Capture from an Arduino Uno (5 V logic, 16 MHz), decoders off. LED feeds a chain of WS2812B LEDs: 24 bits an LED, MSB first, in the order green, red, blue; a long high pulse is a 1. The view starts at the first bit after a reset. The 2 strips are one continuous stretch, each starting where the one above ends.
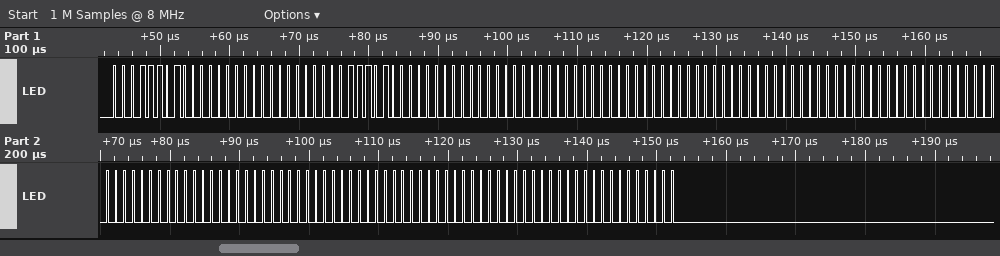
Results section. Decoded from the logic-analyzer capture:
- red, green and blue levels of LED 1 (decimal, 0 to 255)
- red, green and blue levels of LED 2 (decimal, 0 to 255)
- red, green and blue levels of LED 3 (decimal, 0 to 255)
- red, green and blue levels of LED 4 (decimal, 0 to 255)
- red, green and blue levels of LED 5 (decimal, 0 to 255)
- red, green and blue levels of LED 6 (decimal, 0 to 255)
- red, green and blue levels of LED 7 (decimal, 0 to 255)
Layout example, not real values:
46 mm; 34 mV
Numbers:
0, 29, 0; 0, 29, 0; 0, 0, 0; 0, 0, 0; 0, 0, 0; 0, 0, 0; 0, 0, 0
